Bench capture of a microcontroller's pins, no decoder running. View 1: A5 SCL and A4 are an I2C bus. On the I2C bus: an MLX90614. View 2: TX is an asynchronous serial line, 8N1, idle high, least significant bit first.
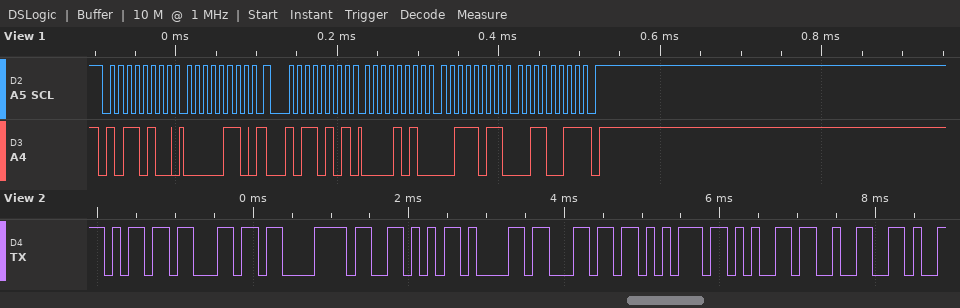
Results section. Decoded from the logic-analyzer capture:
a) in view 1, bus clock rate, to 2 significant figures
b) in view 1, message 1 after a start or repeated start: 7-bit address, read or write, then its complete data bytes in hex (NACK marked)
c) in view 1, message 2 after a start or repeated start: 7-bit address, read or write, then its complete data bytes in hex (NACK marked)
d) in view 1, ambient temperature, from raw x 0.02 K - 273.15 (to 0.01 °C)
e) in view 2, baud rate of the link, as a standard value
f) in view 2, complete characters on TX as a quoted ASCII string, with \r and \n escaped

100 kHz
0x5A write: 06
0x5A read: 0A 3B 33 NACK
29.13 °C
9600 baud
"mlxValue2"
